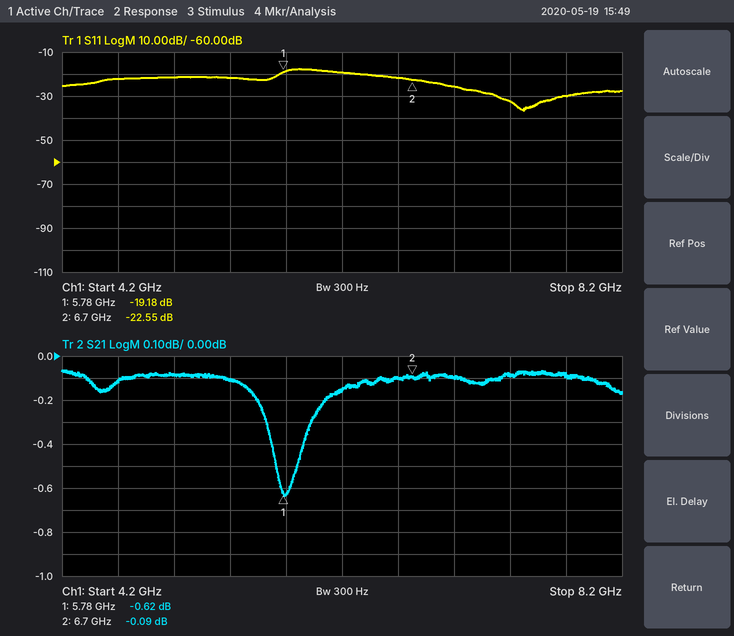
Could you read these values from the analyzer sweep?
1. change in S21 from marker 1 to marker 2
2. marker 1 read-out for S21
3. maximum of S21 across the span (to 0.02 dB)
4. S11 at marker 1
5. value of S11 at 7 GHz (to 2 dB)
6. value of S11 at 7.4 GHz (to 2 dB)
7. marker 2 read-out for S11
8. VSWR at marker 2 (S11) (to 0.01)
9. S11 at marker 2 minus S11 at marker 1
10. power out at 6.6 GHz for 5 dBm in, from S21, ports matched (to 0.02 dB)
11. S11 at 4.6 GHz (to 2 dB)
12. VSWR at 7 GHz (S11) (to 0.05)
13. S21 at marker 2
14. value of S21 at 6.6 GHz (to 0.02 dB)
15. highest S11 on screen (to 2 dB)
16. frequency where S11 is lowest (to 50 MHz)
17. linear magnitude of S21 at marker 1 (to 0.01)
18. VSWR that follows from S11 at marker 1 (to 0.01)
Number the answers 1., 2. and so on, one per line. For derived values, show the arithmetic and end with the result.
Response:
1. -0.09 − (-0.62) = 0.53 dB
2. -0.62 dB
3. -0.06 dB
4. -19.18 dB
5. -26 dB
6. -32 dB
7. -22.55 dB
8. (1 + 0.0746)/(1 − 0.0746) ≈ 1.16
9. -22.55 − (-19.18) = -3.37 dB
10. 5 dBm + (-0.10 dB) = 4.90 dBm
11. -22 dB
12. |Γ| = 10^(-26/20) = 0.0501; VSWR = (1 + 0.0501)/(1 − 0.0501) ≈ 1.11, so 1.10 to the nearest 0.05
13. -0.09 dB
14. -0.10 dB
15. -18 dB
16. 7.50 GHz
17. 10^(-0.62/20) ≈ 0.93
18. (1 + 0.1099)/(1 − 0.1099) ≈ 1.25
